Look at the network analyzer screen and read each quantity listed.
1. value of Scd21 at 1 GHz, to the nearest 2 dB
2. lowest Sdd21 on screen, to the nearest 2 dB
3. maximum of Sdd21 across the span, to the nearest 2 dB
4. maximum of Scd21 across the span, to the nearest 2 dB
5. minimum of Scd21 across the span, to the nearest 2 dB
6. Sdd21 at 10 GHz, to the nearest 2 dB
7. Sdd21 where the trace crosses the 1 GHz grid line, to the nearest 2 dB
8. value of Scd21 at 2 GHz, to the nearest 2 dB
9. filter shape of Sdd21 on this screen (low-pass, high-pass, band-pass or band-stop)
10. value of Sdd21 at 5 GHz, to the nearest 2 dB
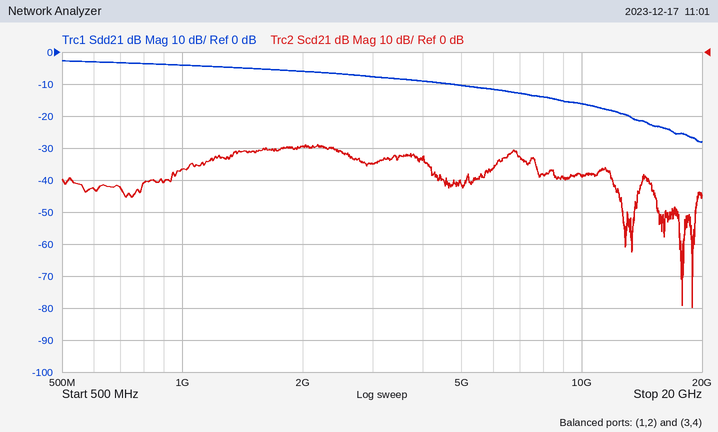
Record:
-36 dB
-28 dB
-2 dB
-28 dB
-80 dB
-16 dB
-4 dB
-30 dB
low-pass
-10 dB
